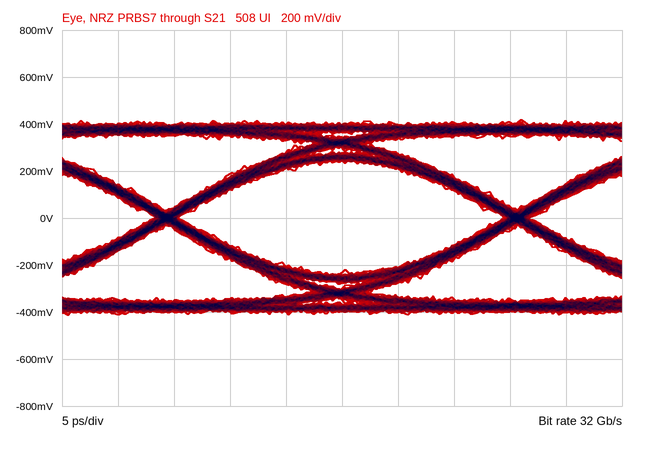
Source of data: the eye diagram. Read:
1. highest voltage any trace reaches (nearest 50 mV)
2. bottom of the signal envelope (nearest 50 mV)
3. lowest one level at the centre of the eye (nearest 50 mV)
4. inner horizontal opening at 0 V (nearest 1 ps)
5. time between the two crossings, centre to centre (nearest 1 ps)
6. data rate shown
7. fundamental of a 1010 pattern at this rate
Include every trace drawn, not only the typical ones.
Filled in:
400 mV
-400 mV
250 mV
29 ps
31 ps
32 Gb/s
16 GHz
